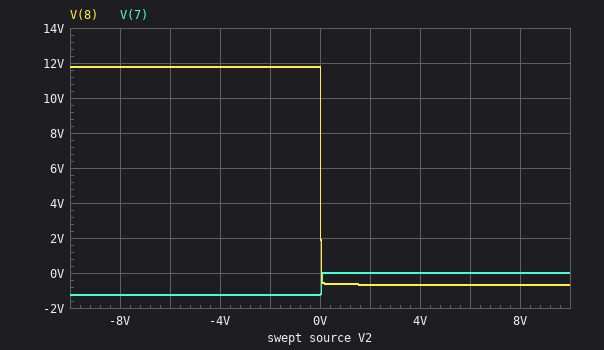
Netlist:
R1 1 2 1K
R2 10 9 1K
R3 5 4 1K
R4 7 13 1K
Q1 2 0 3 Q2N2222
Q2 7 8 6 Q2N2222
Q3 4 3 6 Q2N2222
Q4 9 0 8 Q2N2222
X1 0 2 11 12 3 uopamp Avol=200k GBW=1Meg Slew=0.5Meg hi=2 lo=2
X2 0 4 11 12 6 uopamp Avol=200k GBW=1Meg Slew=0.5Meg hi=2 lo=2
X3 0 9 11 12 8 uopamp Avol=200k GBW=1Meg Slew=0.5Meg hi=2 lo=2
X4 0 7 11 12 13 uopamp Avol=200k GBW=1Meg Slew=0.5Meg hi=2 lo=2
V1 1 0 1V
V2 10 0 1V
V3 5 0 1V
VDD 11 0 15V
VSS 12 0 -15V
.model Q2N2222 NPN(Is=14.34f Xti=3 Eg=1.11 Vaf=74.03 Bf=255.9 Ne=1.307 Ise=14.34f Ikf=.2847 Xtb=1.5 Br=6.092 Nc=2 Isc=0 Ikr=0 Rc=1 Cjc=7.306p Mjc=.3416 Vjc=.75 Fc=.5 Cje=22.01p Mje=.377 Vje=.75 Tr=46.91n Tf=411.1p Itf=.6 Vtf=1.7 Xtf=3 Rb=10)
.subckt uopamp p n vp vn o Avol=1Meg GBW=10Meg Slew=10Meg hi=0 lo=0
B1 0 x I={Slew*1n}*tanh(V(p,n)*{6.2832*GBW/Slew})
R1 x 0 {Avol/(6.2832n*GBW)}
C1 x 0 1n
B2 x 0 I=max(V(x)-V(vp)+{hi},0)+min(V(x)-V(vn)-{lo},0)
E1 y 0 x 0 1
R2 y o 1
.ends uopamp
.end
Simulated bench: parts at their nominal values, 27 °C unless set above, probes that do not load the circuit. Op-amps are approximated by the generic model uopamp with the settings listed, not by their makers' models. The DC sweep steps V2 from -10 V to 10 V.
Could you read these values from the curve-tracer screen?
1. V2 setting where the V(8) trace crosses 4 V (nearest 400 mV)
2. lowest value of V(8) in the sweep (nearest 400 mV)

0 V
-800 mV
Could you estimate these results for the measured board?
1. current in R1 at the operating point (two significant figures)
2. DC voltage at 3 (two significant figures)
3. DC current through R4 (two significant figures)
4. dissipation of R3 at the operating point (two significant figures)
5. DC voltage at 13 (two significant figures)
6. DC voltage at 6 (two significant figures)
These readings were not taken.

1.0 mA
-650 mV
1.0 mA
1.0 mW
1.0 V
-1.3 V
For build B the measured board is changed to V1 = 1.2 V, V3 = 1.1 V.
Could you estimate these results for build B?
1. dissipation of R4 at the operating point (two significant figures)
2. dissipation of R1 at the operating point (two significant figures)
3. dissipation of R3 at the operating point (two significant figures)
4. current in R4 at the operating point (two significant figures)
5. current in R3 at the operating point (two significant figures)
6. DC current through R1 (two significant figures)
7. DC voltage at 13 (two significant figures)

1.7 mW
1.4 mW
1.2 mW
1.3 mA
1.1 mA
1.2 mA
1.3 V
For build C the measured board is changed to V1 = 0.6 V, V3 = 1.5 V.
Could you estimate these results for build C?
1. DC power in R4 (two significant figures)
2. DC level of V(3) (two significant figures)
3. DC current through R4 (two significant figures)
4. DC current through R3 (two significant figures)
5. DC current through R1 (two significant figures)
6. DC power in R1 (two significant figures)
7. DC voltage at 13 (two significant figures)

810 µW
-630 mV
900 µA
1.5 mA
600 µA
360 µW
900 mV
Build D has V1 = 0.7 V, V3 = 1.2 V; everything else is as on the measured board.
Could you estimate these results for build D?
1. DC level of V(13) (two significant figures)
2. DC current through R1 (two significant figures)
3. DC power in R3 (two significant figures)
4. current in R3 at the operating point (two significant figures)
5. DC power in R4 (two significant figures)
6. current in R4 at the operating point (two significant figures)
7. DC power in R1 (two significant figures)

840 mV
700 µA
1.4 mW
1.2 mA
710 µW
840 µA
490 µW
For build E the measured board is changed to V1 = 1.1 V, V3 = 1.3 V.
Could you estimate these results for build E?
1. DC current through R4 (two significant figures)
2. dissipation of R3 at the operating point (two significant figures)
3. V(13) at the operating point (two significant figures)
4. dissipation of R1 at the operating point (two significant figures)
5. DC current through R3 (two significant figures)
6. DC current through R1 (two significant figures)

1.4 mA
1.7 mW
1.4 V
1.2 mW
1.3 mA
1.1 mA
